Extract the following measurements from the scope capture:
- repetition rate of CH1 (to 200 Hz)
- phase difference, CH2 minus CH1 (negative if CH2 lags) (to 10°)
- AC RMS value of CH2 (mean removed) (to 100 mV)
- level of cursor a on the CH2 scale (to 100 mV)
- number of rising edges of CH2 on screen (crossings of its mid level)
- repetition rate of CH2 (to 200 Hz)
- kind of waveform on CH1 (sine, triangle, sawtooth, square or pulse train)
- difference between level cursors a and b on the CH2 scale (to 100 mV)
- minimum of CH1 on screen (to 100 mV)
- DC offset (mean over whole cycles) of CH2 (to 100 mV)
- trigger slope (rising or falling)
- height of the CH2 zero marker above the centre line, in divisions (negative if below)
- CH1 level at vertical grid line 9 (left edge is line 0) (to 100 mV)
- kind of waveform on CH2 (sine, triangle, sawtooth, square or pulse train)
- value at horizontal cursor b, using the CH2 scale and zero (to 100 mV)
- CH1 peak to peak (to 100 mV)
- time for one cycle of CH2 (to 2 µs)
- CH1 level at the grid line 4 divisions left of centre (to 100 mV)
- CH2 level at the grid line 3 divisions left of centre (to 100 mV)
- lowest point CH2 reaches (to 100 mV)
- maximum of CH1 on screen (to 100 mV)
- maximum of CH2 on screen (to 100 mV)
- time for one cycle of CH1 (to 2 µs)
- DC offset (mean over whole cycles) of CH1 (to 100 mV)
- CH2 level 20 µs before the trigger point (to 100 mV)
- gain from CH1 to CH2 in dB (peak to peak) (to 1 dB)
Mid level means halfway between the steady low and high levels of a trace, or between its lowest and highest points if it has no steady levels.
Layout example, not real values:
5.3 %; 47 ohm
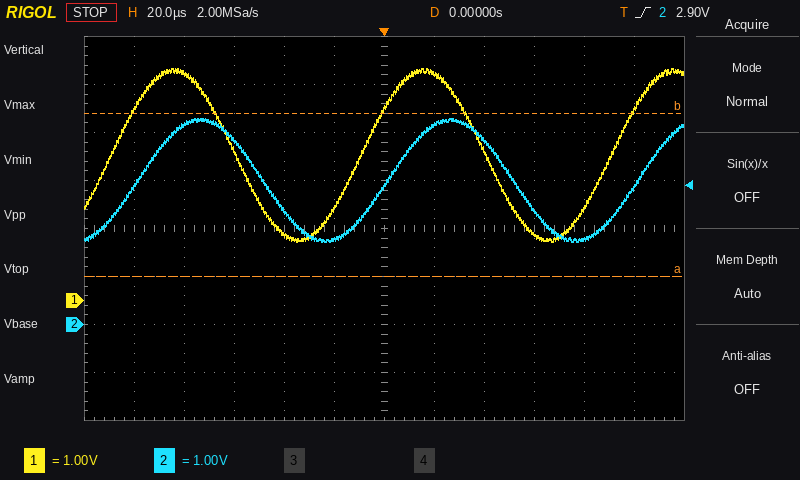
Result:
10.0 kHz; -40°; 900 mV; 1.0 V; 3; 10.0 kHz; sine; 3.4 V; 1.2 V; 3.0 V; rising; -2.0 div; 1.4 V; sine; 4.4 V; 3.6 V; 100 µs; 4.7 V; 3.8 V; 1.7 V; 4.8 V; 4.3 V; 100 µs; 3.0 V; 1.8 V; -3 dB
